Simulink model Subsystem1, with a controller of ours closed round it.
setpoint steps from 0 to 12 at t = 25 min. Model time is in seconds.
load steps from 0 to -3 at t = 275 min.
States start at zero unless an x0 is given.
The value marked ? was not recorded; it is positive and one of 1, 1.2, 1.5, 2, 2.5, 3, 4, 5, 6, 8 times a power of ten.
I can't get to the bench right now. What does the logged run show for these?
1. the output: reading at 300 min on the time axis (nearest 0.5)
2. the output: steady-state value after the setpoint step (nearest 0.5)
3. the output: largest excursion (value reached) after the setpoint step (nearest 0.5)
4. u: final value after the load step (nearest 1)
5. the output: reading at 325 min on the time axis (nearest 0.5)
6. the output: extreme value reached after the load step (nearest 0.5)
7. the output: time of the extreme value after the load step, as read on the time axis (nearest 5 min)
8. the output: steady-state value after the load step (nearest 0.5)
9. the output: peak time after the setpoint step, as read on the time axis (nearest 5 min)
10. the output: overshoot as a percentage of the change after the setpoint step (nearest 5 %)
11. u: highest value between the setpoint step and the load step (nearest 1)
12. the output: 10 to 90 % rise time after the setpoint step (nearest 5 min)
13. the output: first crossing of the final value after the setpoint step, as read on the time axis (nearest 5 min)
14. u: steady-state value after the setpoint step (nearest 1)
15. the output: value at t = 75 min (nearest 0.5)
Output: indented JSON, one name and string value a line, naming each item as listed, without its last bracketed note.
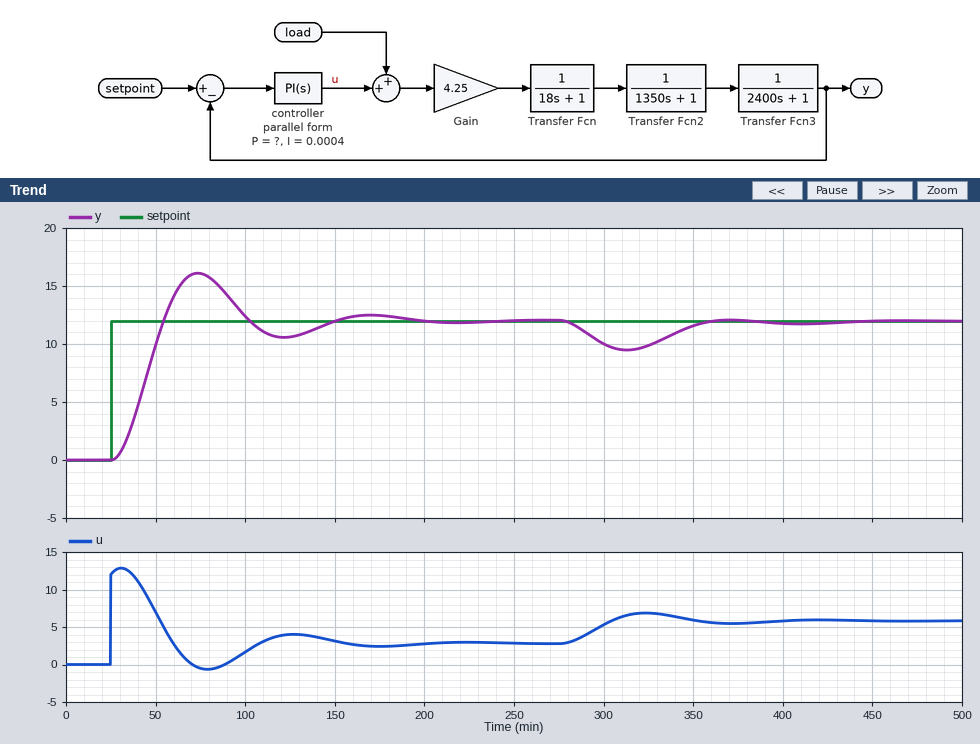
{
  "the output: reading at 300 min on the time axis": "10.0",
  "the output: steady-state value after the setpoint step": "12.0",
  "the output: largest excursion (value reached) after the setpoint step": "16.0",
  "u: final value after the load step": "6",
  "the output: reading at 325 min on the time axis": "10.0",
  "the output: extreme value reached after the load step": "9.5",
  "the output: time of the extreme value after the load step, as read on the time axis": "315 min",
  "the output: steady-state value after the load step": "12.0",
  "the output: peak time after the setpoint step, as read on the time axis": "75 min",
  "the output: overshoot as a percentage of the change after the setpoint step": "35 %",
  "u: highest value between the setpoint step and the load step": "13",
  "the output: 10 to 90 % rise time after the setpoint step": "20 min",
  "the output: first crossing of the final value after the setpoint step, as read on the time axis": "55 min",
  "u: steady-state value after the setpoint step": "3",
  "the output: value at t = 75 min": "16.0"
}
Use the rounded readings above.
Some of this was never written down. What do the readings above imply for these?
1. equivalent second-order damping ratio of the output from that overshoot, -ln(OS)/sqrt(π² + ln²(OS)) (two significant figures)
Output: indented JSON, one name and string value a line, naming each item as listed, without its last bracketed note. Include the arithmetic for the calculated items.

{
  "equivalent second-order damping ratio of the output from that overshoot, -ln(OS)/sqrt(π² + ln²(OS))": "ln(0.35) = -1.050; 1.050 / sqrt(9.870 + 1.102) = 0.32"
}
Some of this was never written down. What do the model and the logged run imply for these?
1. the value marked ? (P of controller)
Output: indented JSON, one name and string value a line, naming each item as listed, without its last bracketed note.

{
  "the value marked ?": "1"
}
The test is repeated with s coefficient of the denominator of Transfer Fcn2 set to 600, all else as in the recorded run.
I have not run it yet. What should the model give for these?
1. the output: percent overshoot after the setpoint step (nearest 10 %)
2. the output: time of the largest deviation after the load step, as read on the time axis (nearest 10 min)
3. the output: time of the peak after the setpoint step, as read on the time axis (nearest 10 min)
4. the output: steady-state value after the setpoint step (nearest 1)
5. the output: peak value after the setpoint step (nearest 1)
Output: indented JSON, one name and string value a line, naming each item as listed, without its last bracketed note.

{
  "the output: percent overshoot after the setpoint step": "20 %",
  "the output: time of the largest deviation after the load step, as read on the time axis": "300 min",
  "the output: time of the peak after the setpoint step, as read on the time axis": "60 min",
  "the output: steady-state value after the setpoint step": "12",
  "the output: peak value after the setpoint step": "14"
}
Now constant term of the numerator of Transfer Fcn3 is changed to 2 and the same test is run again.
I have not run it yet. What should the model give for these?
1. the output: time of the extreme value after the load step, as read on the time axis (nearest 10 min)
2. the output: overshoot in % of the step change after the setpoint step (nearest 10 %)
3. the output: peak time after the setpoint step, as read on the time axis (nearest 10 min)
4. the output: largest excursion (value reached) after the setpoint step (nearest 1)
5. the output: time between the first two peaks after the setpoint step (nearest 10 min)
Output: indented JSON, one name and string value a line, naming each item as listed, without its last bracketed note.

{
  "the output: time of the extreme value after the load step, as read on the time axis": "300 min",
  "the output: overshoot in % of the step change after the setpoint step": "50 %",
  "the output: peak time after the setpoint step, as read on the time axis": "60 min",
  "the output: largest excursion (value reached) after the setpoint step": "18",
  "the output: time between the first two peaks after the setpoint step": "70 min"
}
